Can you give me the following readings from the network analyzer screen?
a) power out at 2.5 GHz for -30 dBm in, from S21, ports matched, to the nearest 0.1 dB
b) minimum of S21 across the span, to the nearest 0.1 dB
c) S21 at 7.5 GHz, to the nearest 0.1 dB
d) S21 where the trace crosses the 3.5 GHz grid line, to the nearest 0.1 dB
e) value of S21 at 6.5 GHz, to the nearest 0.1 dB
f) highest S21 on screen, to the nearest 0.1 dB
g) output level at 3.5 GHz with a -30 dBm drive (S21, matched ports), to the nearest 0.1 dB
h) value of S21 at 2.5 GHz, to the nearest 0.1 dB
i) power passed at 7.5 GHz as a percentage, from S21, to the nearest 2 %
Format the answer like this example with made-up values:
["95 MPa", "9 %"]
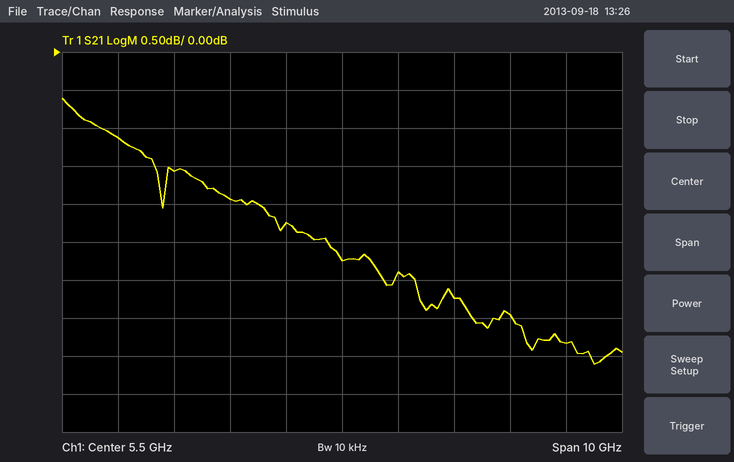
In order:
["-31.6 dBm", "-4.1 dB", "-3.2 dB", "-1.9 dB", "-2.9 dB", "-0.6 dB", "-31.9 dBm", "-1.6 dB", "48 %"]
